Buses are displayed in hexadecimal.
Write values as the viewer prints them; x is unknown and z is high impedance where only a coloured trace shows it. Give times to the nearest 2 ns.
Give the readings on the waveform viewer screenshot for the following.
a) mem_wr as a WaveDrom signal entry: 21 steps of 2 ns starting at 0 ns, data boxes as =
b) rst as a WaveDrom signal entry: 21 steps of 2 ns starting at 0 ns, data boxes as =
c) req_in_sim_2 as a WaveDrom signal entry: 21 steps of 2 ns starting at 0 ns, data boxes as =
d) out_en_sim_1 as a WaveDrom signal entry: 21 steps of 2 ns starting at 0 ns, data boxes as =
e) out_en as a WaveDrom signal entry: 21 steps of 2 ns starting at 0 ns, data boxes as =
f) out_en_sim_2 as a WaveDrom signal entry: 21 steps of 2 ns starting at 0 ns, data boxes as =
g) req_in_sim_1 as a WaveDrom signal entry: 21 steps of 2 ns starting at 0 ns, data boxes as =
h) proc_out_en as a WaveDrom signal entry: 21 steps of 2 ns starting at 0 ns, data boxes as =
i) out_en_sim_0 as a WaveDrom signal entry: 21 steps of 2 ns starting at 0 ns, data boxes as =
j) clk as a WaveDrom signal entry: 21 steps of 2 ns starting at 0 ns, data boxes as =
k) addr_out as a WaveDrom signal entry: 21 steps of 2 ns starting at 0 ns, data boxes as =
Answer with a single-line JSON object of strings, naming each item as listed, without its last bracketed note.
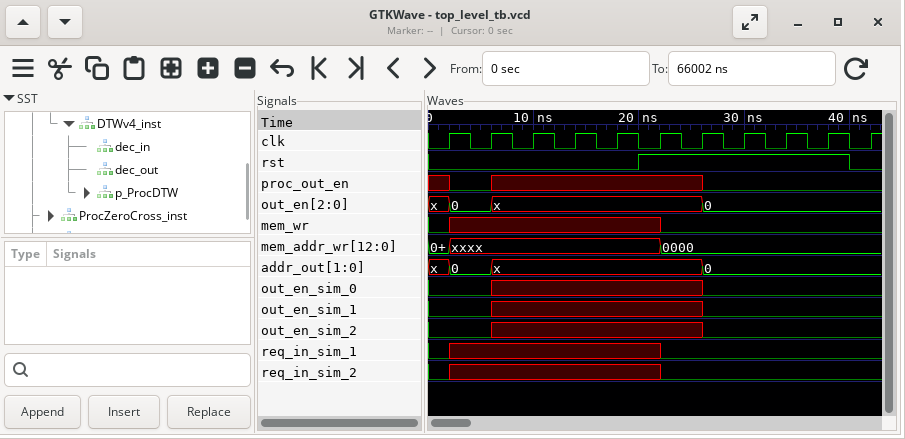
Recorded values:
{"mem_wr as a WaveDrom signal entry: 21 steps of 2 ns starting at 0 ns, data boxes as =": "{name: 'mem_wr', wave: '0x.........0.........'}", "rst as a WaveDrom signal entry: 21 steps of 2 ns starting at 0 ns, data boxes as =": "{name: 'rst', wave: '0.........1.........0'}", "req_in_sim_2 as a WaveDrom signal entry: 21 steps of 2 ns starting at 0 ns, data boxes as =": "{name: 'req_in_sim_2', wave: '0x.........0.........'}", "out_en_sim_1 as a WaveDrom signal entry: 21 steps of 2 ns starting at 0 ns, data boxes as =": "{name: 'out_en_sim_1', wave: '0..x.........0.......'}", "out_en as a WaveDrom signal entry: 21 steps of 2 ns starting at 0 ns, data boxes as =": "{name: 'out_en', wave: 'x=.x.........=.......', data: '0 0'}", "out_en_sim_2 as a WaveDrom signal entry: 21 steps of 2 ns starting at 0 ns, data boxes as =": "{name: 'out_en_sim_2', wave: '0..x.........0.......'}", "req_in_sim_1 as a WaveDrom signal entry: 21 steps of 2 ns starting at 0 ns, data boxes as =": "{name: 'req_in_sim_1', wave: '0x.........0.........'}", "proc_out_en as a WaveDrom signal entry: 21 steps of 2 ns starting at 0 ns, data boxes as =": "{name: 'proc_out_en', wave: 'x0.x.........0.......'}", "out_en_sim_0 as a WaveDrom signal entry: 21 steps of 2 ns starting at 0 ns, data boxes as =": "{name: 'out_en_sim_0', wave: '0..x.........0.......'}", "clk as a WaveDrom signal entry: 21 steps of 2 ns starting at 0 ns, data boxes as =": "{name: 'clk', wave: '010101010101010101010'}", "addr_out as a WaveDrom signal entry: 21 steps of 2 ns starting at 0 ns, data boxes as =": "{name: 'addr_out', wave: 'x=.x.........=.......', data: '0 0'}"}
